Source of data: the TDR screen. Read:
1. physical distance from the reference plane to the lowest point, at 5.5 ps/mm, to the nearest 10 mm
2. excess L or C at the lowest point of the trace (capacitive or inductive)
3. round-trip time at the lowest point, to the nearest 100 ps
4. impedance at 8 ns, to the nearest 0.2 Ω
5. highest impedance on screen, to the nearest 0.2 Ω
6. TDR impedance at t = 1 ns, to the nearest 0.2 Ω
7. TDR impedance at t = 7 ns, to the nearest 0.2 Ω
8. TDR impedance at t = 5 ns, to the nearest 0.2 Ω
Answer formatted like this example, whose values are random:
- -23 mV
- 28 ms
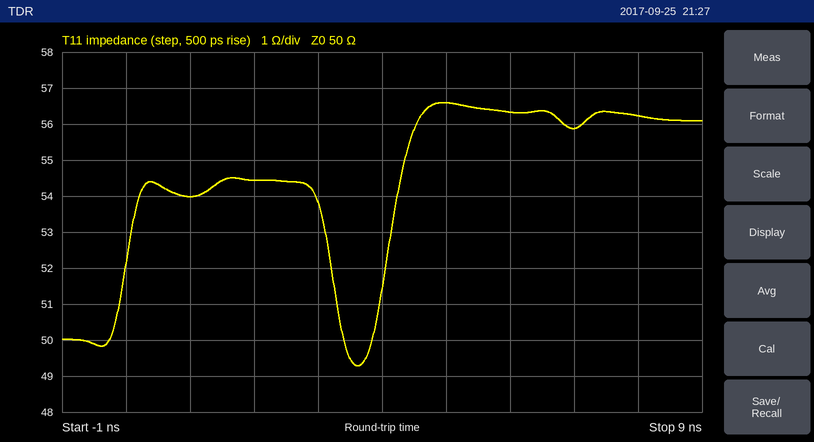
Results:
- 330 mm
- capacitive
- 3.6 ns
- 56.2 Ω
- 56.6 Ω
- 54.0 Ω
- 55.8 Ω
- 56.6 Ω
